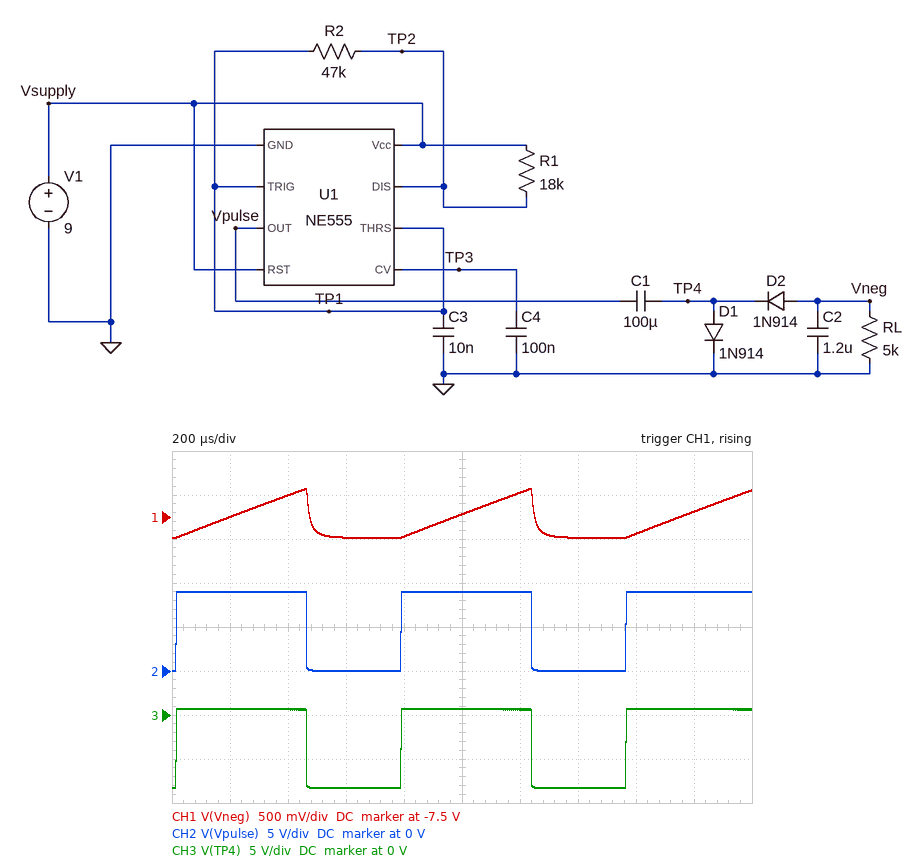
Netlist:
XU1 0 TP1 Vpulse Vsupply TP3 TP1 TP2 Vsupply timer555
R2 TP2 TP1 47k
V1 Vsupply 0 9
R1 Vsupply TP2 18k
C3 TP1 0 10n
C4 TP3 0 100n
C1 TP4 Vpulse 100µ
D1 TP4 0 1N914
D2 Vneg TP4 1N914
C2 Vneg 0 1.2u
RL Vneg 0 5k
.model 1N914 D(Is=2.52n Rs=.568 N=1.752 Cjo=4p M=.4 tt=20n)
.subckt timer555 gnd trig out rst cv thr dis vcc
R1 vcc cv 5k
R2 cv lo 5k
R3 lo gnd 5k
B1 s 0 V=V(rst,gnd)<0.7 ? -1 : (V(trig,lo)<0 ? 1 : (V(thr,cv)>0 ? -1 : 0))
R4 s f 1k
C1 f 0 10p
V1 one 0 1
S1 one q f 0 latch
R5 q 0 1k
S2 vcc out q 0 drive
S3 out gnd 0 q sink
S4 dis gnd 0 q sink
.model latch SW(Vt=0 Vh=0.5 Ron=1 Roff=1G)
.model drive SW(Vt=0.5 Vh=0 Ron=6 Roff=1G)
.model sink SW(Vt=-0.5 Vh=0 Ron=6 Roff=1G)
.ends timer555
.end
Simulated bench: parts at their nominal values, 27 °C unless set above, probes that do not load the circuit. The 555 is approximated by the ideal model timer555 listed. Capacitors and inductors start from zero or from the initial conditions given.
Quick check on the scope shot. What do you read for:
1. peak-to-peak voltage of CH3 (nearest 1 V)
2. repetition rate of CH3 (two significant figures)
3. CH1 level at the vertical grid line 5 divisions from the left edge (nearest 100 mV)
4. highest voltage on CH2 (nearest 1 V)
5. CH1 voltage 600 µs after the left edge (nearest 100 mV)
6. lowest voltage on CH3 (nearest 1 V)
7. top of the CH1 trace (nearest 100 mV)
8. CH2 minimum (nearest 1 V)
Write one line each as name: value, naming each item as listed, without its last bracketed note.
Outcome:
peak-to-peak voltage of CH3: 9 V
repetition rate of CH3: 1.3 kHz
CH1 level at the vertical grid line 5 divisions from the left edge: -7.5 V
highest voltage on CH2: 9 V
CH1 voltage 600 µs after the left edge: -7.7 V
lowest voltage on CH3: -8 V
top of the CH1 trace: -7.2 V
CH2 minimum: 0 V
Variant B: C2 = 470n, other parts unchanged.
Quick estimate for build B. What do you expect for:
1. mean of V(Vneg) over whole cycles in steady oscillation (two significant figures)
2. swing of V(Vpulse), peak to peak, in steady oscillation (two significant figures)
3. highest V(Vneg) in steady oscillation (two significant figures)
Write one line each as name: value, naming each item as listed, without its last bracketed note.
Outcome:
mean of V(Vneg) over whole cycles in steady oscillation: -7.3 V
swing of V(Vpulse), peak to peak, in steady oscillation: 9.0 V
highest V(Vneg) in steady oscillation: -6.4 V
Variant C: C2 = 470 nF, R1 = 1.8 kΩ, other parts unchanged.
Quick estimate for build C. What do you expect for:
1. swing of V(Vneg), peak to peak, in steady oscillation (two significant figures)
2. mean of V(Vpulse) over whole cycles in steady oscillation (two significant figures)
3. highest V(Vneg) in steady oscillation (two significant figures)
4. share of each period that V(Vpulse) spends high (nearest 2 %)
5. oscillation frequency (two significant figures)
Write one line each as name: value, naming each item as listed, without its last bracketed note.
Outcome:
swing of V(Vneg), peak to peak, in steady oscillation: 1.0 V
mean of V(Vpulse) over whole cycles in steady oscillation: 4.6 V
highest V(Vneg) in steady oscillation: -6.7 V
share of each period that V(Vpulse) spends high: 50 %
oscillation frequency: 1.5 kHz
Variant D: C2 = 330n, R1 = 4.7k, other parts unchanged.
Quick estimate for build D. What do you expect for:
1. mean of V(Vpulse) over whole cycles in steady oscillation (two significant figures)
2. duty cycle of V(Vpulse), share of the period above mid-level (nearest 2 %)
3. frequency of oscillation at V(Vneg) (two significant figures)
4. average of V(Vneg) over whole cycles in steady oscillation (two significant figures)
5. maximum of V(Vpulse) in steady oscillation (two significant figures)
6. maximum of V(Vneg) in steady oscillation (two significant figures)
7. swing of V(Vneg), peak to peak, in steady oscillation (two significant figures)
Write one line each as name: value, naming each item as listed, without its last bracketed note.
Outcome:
mean of V(Vpulse) over whole cycles in steady oscillation: 4.7 V
duty cycle of V(Vpulse), share of the period above mid-level: 52 %
frequency of oscillation at V(Vneg): 1.5 kHz
average of V(Vneg) over whole cycles in steady oscillation: -7.3 V
maximum of V(Vpulse) in steady oscillation: 9.0 V
maximum of V(Vneg) in steady oscillation: -6.2 V
swing of V(Vneg), peak to peak, in steady oscillation: 1.5 V
